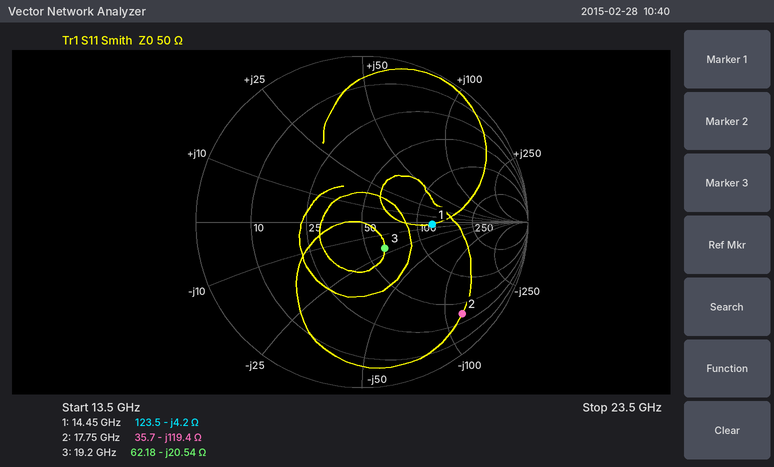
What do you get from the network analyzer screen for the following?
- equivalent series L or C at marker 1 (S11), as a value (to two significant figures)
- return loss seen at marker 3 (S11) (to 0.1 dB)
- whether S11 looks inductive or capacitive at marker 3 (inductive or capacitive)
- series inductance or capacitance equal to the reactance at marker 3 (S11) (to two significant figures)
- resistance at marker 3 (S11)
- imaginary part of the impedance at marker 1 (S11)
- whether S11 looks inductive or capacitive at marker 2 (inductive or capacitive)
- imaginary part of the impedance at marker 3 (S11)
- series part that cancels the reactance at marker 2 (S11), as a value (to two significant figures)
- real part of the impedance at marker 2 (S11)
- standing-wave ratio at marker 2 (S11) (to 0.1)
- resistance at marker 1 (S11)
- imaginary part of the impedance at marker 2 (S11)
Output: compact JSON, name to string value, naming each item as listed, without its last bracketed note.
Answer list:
{"equivalent series L or C at marker 1 (S11), as a value": "2.6 pF", "return loss seen at marker 3 (S11)": "13.6 dB", "whether S11 looks inductive or capacitive at marker 3": "capacitive", "series inductance or capacitance equal to the reactance at marker 3 (S11)": "400 fF", "resistance at marker 3": "62.18 Ω", "imaginary part of the impedance at marker 1": "-4.2 Ω", "whether S11 looks inductive or capacitive at marker 2": "capacitive", "imaginary part of the impedance at marker 3": "-20.54 Ω", "series part that cancels the reactance at marker 2 (S11), as a value": "1.1 nH", "real part of the impedance at marker 2": "35.7 Ω", "standing-wave ratio at marker 2 (S11)": "10.0", "resistance at marker 1": "123.5 Ω", "imaginary part of the impedance at marker 2": "-119.4 Ω"}
